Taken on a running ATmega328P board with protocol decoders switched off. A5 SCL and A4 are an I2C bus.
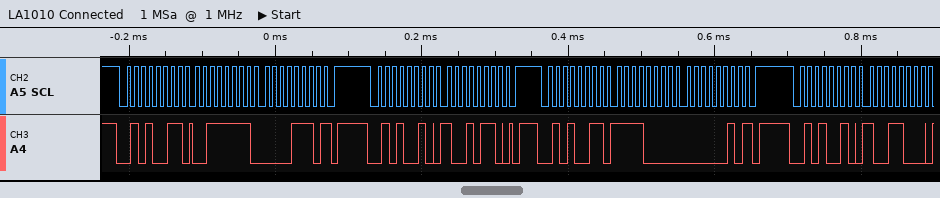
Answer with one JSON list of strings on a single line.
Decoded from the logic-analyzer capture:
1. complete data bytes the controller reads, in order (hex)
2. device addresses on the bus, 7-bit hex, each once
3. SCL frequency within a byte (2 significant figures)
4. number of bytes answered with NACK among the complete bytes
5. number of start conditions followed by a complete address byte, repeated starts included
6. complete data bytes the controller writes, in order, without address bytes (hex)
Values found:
["3F 0E F0 02", "0x29", "100 kHz", "2", "4", "96 98"]
